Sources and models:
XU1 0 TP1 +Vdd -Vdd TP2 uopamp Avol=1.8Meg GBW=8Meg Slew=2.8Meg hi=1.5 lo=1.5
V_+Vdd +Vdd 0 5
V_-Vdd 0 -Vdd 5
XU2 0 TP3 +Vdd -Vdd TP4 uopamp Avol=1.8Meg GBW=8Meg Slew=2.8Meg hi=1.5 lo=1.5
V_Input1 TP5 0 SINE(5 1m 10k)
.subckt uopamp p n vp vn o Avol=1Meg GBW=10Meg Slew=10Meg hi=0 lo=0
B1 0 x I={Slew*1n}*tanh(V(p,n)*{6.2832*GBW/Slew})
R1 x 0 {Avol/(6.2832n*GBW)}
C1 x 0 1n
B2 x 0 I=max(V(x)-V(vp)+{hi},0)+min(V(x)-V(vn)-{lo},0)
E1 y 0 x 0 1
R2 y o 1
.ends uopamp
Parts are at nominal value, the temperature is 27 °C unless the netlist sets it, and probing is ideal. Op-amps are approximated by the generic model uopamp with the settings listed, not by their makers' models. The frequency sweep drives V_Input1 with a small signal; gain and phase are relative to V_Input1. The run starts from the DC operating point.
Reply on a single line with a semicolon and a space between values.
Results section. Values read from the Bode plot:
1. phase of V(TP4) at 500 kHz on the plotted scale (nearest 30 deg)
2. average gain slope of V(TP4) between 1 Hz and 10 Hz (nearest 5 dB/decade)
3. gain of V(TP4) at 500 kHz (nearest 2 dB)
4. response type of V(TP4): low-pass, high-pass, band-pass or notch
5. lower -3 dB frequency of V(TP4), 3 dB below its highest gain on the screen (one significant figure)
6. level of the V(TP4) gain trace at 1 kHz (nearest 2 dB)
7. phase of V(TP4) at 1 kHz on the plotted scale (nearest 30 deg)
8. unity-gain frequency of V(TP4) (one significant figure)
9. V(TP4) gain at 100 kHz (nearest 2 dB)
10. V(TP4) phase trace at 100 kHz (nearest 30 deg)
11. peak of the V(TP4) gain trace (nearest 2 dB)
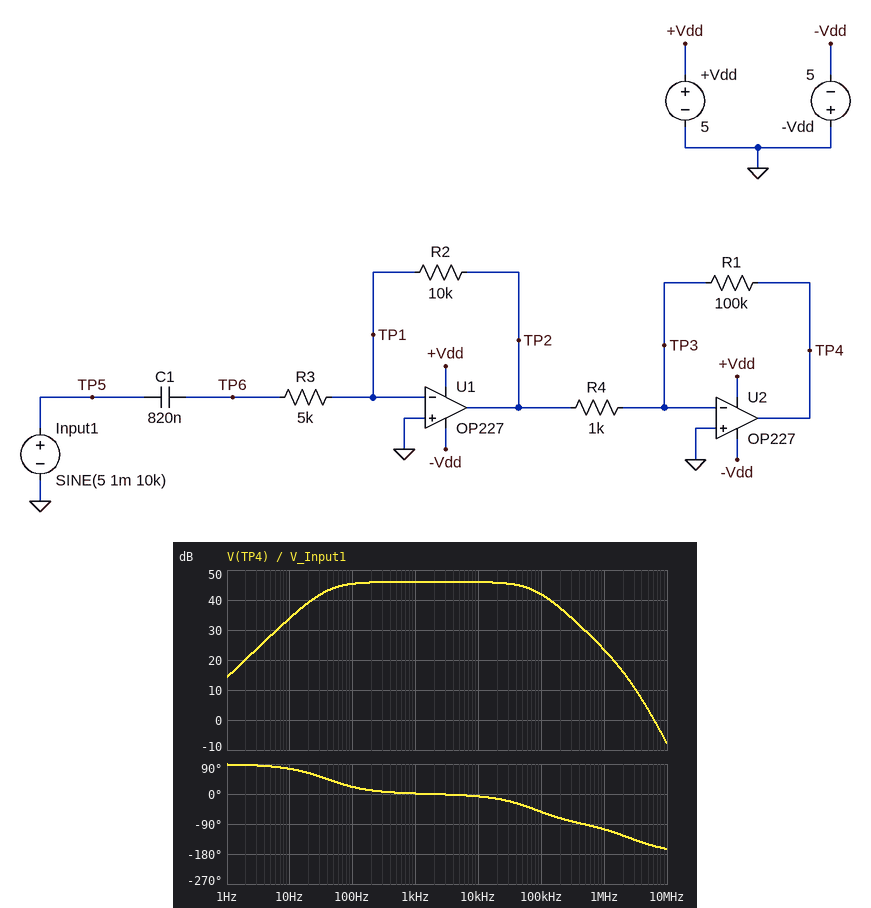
-90 deg; 20 dB/decade; 30 dB; band-pass; 40 Hz; 46 dB; 0 deg; 6 MHz; 42 dB; -60 deg; 46 dB
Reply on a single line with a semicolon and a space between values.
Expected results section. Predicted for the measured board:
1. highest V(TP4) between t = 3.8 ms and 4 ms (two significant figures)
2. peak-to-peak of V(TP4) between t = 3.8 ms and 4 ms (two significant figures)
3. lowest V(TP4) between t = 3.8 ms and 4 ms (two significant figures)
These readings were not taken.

200 mV; 400 mV; -200 mV
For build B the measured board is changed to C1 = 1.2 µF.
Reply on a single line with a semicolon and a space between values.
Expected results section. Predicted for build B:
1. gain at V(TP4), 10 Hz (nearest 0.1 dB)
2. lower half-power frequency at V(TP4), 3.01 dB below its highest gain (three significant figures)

37.0 dB; 26.5 Hz
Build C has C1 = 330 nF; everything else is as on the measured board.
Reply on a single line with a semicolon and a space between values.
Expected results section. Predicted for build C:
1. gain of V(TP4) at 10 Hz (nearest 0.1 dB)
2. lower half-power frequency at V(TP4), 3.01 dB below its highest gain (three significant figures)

26.3 dB; 96.2 Hz
